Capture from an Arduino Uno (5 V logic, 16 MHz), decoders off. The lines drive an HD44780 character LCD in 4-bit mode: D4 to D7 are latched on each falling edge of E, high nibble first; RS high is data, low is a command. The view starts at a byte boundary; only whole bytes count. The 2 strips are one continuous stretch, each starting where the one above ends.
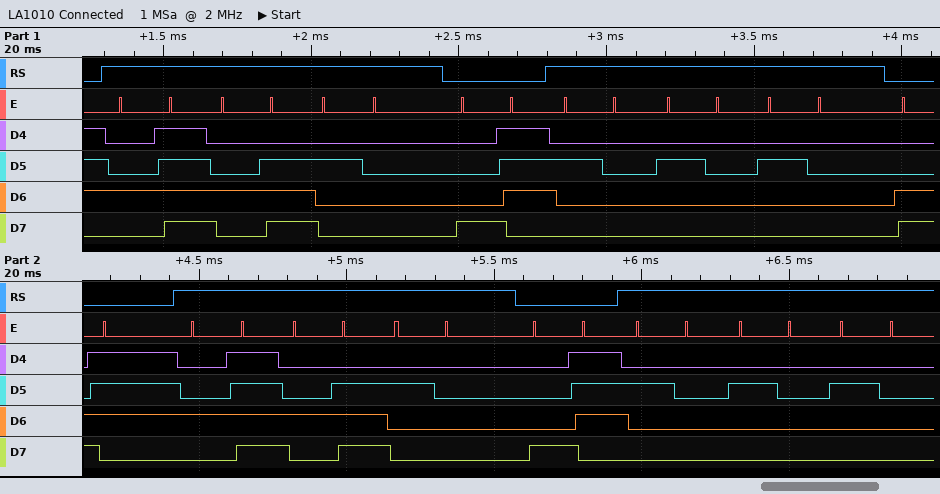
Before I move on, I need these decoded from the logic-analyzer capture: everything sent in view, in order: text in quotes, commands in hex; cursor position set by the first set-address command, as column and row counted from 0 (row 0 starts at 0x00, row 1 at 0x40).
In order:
"ON " 0x87 "   " 0xC7 "ON " 0x87 "   "
column 7, row 0
